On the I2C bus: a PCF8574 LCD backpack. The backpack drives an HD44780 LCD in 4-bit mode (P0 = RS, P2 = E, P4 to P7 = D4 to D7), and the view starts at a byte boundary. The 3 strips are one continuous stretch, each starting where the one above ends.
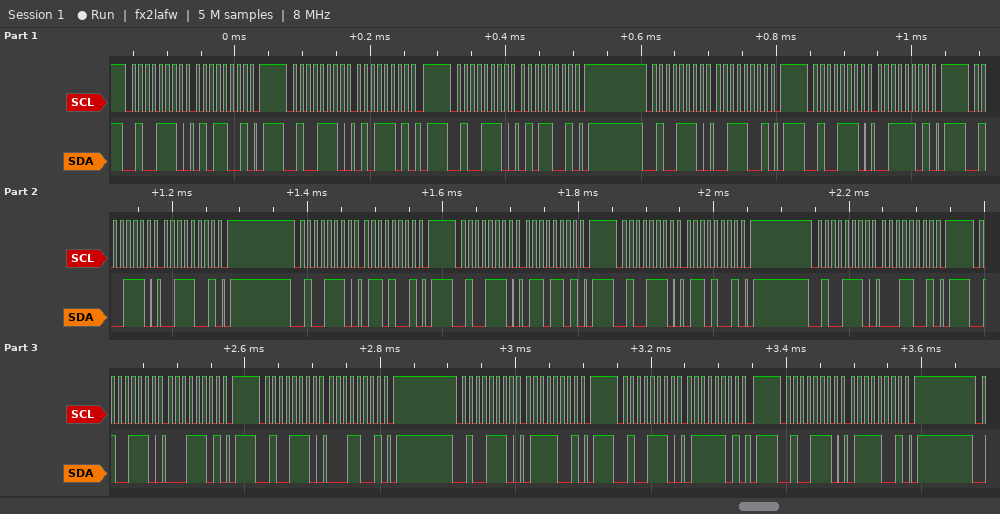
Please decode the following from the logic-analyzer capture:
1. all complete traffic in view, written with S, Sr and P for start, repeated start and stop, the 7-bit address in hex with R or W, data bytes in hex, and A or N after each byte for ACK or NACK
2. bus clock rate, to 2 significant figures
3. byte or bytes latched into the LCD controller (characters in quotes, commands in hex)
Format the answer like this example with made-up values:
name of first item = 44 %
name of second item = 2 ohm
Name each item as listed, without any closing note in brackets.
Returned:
all complete traffic in view, written with S, Sr and P for start, repeated start and stop, the 7-bit address in hex with R or W, data bytes in hex, and A or N after each byte for ACK or NACK = S 27W A 59 A P S 27W A 5D A P S 27W A 59 A P S 27W A 39 A P S 27W A 3D A P S 27W A 39 A P S 27W A 69 A P S 27W A 6D A P S 27W A 69 A P S 27W A 19 A P S 27W A 1D A P S 27W A 19 A P S 27W A 79 A P S 27W A 7D A P S 27W A 79 A P
bus clock rate, to 2 significant figures = 100 kHz
byte or bytes latched into the LCD controller = 'S' 'a'
